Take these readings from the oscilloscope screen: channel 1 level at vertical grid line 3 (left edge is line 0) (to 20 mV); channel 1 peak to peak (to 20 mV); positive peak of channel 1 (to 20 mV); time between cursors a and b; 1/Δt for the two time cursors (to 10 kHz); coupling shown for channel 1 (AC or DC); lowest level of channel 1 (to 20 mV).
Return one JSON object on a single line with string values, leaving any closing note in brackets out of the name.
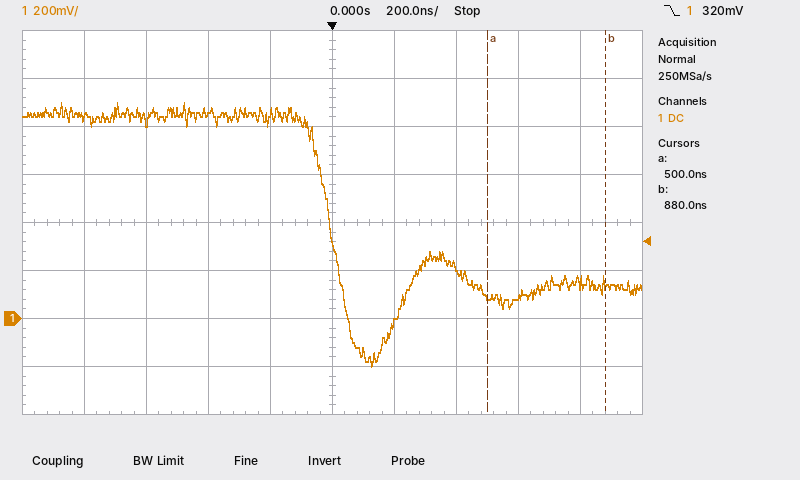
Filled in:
{"channel 1 level at vertical grid line 3 (left edge is line 0)": "860 mV", "channel 1 peak to peak": "1.10 V", "positive peak of channel 1": "900 mV", "time between cursors a and b": "380 ns", "1/Δt for the two time cursors": "2.63 MHz", "coupling shown for channel 1": "DC", "lowest level of channel 1": "-200 mV"}
